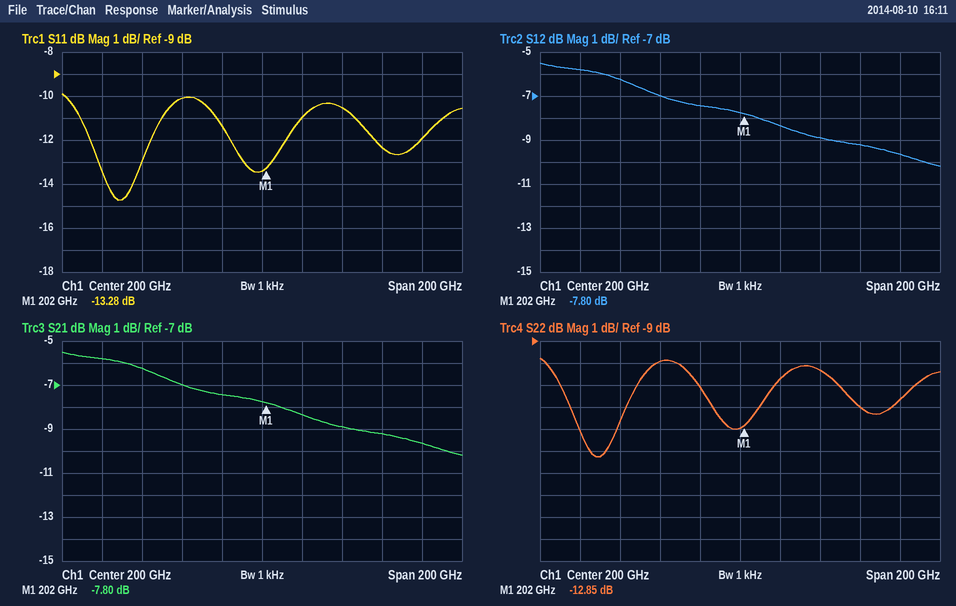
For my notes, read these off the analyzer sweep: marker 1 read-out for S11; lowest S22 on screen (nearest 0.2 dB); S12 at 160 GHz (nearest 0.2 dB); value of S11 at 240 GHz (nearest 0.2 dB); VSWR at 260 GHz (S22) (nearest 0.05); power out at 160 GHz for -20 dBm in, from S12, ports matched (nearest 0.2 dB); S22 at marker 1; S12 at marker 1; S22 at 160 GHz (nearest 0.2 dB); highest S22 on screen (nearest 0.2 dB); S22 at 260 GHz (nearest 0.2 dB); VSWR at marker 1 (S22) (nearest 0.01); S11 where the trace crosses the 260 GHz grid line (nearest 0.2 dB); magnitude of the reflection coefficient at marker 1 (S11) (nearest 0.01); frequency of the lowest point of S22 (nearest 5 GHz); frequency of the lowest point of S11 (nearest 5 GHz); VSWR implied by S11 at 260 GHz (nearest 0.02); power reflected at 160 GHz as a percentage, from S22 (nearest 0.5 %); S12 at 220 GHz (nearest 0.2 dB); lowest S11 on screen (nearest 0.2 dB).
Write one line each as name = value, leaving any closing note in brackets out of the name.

marker 1 read-out for S11 = -13.28 dB
lowest S22 on screen = -14.2 dB
S12 at 160 GHz = -7.0 dB
value of S11 at 240 GHz = -10.6 dB
VSWR at 260 GHz (S22) = 1.65
power out at 160 GHz for -20 dBm in, from S12, ports matched = -27.0 dBm
S22 at marker 1 = -12.85 dB
S12 at marker 1 = -7.80 dB
S22 at 160 GHz = -10.0 dB
highest S22 on screen = -9.8 dB
S22 at 260 GHz = -12.0 dB
VSWR at marker 1 (S22) = 1.59
S11 where the trace crosses the 260 GHz grid line = -12.4 dB
magnitude of the reflection coefficient at marker 1 (S11) = 0.22
frequency of the lowest point of S22 = 130 GHz
frequency of the lowest point of S11 = 130 GHz
VSWR implied by S11 at 260 GHz = 1.64
power reflected at 160 GHz as a percentage, from S22 = 10.0 %
S12 at 220 GHz = -8.4 dB
lowest S11 on screen = -14.8 dB
